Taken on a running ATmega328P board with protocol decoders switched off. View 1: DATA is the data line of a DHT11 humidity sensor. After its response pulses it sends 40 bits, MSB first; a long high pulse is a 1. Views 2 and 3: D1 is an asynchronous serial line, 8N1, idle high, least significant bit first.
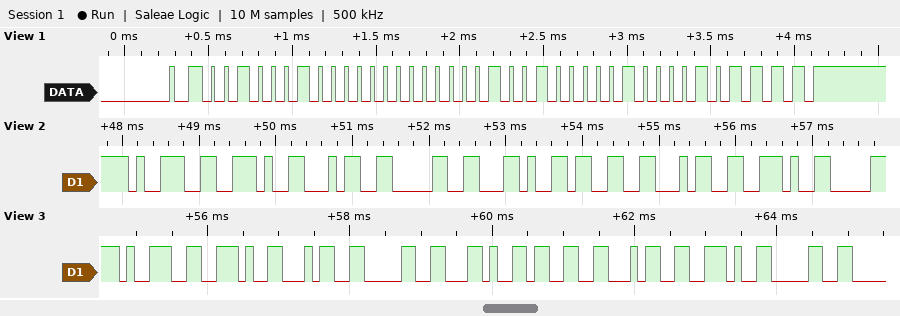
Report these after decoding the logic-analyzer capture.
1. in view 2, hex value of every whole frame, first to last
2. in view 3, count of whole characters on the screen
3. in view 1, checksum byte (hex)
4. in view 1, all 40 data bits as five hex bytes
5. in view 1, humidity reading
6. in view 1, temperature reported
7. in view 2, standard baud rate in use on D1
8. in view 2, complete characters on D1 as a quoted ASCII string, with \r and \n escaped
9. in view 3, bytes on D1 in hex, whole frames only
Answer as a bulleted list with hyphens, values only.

- 39 2E 34 30 2C 33 34 2E
- 9
- 0x2F
- 22 00 09 04 2F
- 34 %
- 9.4 °C
- 9600 baud
- "9.40,34."
- 0x39 0x2E 0x34 0x30 0x2C 0x33 0x34 0x2E 0x30
